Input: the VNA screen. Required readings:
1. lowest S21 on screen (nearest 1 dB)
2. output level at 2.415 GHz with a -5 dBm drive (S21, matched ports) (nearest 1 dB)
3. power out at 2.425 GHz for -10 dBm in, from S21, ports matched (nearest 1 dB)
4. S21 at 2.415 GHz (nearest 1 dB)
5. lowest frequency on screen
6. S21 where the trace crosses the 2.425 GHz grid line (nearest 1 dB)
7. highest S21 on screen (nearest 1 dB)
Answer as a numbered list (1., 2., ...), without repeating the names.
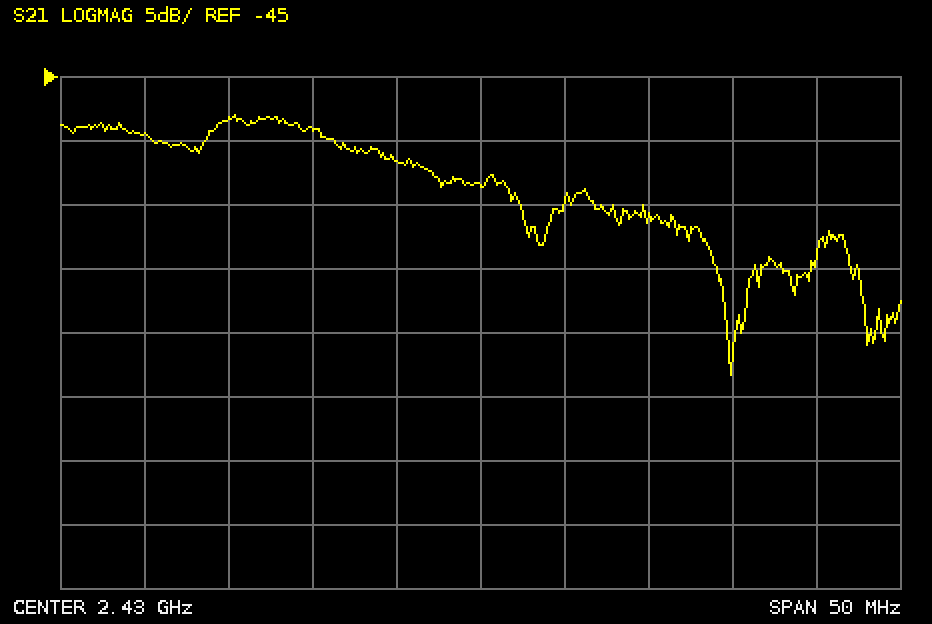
1. -68 dB
2. -53 dBm
3. -62 dBm
4. -48 dB
5. 2.405 GHz
6. -52 dB
7. -48 dB
